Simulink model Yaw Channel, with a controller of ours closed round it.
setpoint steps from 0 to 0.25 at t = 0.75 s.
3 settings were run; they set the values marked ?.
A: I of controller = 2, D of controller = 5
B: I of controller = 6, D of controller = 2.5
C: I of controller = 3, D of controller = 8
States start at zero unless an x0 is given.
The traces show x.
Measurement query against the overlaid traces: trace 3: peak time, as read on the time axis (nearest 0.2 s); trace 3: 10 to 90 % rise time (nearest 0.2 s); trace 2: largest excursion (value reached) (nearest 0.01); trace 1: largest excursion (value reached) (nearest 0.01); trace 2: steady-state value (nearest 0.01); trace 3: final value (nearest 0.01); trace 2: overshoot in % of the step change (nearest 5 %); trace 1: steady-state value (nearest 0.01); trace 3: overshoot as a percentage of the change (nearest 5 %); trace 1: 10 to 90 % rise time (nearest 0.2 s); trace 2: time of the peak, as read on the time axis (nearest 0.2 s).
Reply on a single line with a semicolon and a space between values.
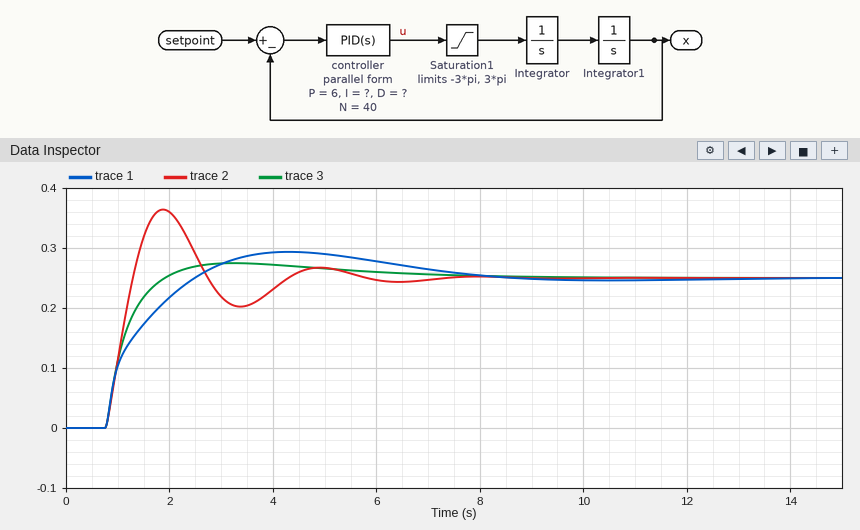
3.2 s; 0.8 s; 0.36; 0.29; 0.25; 0.25; 45 %; 0.25; 10 %; 1.2 s; 1.8 s
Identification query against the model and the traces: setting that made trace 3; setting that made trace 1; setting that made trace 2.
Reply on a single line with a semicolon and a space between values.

A; C; B
